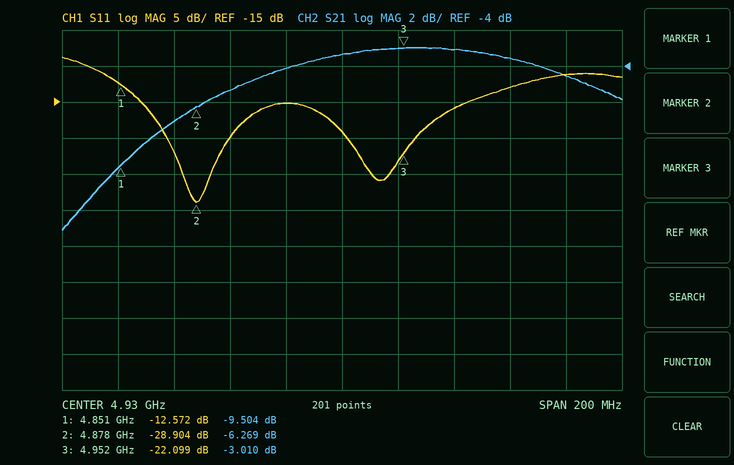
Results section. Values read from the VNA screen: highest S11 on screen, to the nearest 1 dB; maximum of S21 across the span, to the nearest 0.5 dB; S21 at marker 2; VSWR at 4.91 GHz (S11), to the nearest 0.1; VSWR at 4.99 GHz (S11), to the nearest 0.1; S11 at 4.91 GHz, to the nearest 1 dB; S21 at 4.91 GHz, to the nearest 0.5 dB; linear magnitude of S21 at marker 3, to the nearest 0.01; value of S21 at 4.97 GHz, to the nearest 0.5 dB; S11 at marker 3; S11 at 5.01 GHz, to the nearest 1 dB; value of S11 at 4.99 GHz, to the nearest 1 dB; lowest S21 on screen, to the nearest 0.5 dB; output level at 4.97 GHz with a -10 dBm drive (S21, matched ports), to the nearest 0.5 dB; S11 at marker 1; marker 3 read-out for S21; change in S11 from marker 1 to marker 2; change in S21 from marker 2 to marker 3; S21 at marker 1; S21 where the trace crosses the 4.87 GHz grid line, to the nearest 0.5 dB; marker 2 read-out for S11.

-9 dB
-3.0 dB
-6.269 dB
1.4
1.6
-15 dB
-4.0 dB
0.71
-3.0 dB
-22.099 dB
-11 dB
-13 dB
-13.0 dB
-13.0 dBm
-12.572 dB
-3.010 dB
-16.332 dB
3.259 dB
-9.504 dB
-7.0 dB
-28.904 dB
